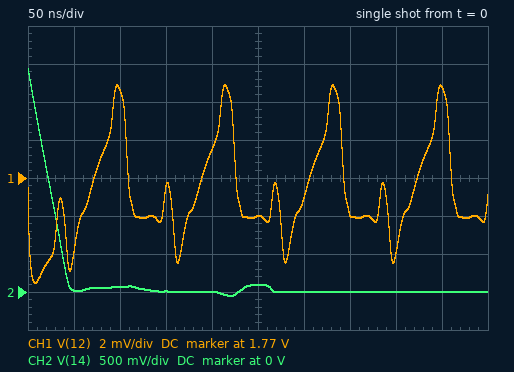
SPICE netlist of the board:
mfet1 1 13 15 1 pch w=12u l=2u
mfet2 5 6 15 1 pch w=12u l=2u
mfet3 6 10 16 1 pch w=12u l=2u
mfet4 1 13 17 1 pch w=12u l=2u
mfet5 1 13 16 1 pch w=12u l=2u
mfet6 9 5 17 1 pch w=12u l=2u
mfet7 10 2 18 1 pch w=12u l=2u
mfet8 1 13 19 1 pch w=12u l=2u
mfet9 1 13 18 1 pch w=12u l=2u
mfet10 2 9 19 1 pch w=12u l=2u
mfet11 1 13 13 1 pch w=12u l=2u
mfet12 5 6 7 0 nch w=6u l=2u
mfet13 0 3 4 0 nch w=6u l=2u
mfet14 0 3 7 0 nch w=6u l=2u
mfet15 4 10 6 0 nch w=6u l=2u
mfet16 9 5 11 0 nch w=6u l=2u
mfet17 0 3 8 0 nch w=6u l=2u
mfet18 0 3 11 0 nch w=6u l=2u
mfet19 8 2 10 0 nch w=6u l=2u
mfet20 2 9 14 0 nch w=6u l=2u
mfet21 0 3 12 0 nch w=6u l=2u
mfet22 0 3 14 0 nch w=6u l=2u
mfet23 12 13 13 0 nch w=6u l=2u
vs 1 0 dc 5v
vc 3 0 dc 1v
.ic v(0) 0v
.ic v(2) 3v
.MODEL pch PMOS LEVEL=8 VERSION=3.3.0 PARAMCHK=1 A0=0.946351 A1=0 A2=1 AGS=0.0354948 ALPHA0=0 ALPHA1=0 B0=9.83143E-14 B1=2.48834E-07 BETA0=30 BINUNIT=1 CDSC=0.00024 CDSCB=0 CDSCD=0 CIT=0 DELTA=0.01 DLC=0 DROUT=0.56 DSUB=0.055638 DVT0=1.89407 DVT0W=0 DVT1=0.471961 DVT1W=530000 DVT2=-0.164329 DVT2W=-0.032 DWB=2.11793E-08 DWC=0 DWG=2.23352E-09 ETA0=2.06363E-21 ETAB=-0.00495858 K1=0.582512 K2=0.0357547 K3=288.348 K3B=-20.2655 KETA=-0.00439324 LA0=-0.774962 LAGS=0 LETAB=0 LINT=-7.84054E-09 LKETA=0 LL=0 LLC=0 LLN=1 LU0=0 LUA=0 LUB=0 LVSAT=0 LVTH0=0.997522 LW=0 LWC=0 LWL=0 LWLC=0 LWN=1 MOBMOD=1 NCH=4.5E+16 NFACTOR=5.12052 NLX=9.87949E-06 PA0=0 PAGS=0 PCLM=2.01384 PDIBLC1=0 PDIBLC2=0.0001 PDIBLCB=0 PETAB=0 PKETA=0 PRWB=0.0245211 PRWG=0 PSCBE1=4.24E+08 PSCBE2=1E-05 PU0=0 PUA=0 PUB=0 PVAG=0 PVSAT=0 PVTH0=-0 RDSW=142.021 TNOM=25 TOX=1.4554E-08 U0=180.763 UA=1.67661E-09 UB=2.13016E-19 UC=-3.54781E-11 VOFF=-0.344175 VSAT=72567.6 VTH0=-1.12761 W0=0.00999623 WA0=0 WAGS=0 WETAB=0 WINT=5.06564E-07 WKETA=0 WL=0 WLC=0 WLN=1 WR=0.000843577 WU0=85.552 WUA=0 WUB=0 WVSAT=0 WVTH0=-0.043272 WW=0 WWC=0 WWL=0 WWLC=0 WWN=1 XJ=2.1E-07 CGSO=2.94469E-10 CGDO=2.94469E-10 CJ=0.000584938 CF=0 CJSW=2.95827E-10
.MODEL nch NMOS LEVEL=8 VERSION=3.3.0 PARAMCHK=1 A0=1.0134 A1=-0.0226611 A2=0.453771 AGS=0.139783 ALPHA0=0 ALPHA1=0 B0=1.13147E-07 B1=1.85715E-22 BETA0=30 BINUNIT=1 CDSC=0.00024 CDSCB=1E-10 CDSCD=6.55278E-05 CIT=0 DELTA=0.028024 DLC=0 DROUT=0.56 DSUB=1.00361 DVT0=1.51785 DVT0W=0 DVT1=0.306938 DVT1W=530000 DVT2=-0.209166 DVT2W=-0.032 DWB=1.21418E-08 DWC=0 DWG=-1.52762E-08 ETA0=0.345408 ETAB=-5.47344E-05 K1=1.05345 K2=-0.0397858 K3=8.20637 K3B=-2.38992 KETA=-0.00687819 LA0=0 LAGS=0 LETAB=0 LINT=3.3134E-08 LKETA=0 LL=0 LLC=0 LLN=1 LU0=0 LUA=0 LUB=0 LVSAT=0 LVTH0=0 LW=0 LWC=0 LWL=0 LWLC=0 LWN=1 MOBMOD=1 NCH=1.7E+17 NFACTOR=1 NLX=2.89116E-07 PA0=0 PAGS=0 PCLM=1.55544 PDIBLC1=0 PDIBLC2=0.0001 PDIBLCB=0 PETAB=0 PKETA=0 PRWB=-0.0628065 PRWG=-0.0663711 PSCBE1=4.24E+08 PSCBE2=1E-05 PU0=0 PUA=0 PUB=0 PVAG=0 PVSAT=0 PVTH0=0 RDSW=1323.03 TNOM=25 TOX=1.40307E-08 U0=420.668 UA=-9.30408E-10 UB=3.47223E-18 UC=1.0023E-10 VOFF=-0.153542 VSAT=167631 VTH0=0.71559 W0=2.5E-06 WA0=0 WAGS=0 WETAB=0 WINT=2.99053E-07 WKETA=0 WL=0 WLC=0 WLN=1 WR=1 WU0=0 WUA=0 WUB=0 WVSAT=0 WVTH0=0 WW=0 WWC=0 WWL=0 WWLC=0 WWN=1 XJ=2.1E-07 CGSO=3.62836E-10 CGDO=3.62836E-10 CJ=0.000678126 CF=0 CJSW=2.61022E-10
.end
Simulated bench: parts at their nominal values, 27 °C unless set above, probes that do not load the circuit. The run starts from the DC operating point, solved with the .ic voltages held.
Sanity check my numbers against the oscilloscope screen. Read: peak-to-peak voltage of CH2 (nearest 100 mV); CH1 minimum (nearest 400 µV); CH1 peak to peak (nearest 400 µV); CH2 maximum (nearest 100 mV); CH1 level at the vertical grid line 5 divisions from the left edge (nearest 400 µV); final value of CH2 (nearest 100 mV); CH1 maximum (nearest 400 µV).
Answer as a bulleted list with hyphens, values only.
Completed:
- 3.0 V
- 1.7644 V
- 10.4 mV
- 2.9 V
- 1.7680 V
- 0 V
- 1.7748 V
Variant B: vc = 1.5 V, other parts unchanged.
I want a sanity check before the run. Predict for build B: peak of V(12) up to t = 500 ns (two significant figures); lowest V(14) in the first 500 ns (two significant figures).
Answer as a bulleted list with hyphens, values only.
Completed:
- 960 mV
- -120 mV
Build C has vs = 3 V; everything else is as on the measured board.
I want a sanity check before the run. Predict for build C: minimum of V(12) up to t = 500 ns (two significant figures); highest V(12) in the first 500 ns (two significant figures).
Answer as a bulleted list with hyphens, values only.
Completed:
- 280 mV
- 290 mV
